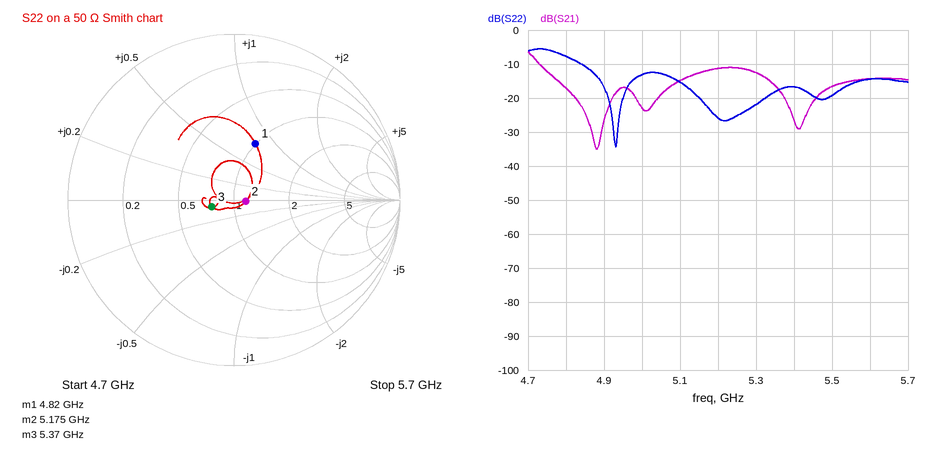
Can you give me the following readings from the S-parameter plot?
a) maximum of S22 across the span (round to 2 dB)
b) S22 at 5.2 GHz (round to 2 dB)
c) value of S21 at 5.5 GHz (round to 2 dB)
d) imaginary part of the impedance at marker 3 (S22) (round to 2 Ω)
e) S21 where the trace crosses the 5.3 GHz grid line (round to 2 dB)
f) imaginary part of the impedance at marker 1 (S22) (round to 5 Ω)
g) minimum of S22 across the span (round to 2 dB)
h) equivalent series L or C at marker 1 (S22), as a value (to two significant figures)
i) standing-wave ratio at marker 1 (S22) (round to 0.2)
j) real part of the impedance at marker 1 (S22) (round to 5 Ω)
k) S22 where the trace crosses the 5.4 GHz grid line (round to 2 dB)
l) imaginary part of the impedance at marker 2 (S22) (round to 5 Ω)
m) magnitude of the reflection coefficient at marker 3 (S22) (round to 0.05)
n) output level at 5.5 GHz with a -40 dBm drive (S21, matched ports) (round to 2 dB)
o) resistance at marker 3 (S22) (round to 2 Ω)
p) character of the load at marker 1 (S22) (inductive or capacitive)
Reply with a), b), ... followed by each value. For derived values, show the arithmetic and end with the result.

a) -6 dB
b) -26 dB
c) -16 dB
d) -4 Ω
e) -12 dB
f) +40 Ω
g) -34 dB
h) L = 40 Ω/(2π × 4.82 GHz) ≈ 1.3 nH
i) 2.2
j) 50 Ω
k) -16 dB
l) 0 Ω
m) 0.15
n) -40 dBm + (-16 dB) = -56 dBm
o) 38 Ω
p) inductive
